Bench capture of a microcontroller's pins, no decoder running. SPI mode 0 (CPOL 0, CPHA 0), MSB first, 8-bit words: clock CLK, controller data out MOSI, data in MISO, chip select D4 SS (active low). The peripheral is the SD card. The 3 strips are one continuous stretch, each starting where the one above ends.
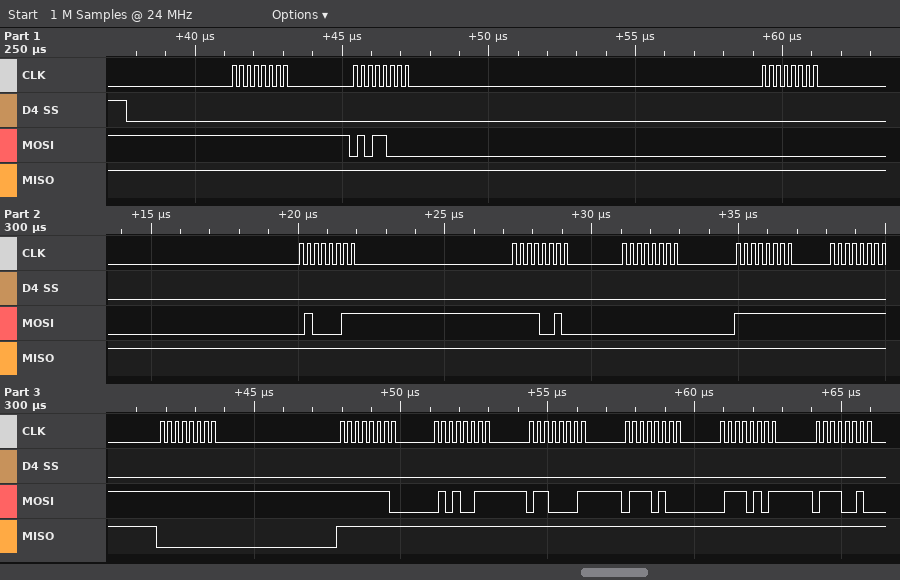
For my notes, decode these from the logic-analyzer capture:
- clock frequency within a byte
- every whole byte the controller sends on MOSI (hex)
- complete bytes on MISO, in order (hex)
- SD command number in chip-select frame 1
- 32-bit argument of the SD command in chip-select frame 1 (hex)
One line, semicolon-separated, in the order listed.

4 MHz; FF 58 00 43 F2 00 FF FF FF FE 53 61 74 75 72; FF FF FF FF FF FF FF FF 00 FF FF FF FF FF FF; CMD24; 0x0043F200
